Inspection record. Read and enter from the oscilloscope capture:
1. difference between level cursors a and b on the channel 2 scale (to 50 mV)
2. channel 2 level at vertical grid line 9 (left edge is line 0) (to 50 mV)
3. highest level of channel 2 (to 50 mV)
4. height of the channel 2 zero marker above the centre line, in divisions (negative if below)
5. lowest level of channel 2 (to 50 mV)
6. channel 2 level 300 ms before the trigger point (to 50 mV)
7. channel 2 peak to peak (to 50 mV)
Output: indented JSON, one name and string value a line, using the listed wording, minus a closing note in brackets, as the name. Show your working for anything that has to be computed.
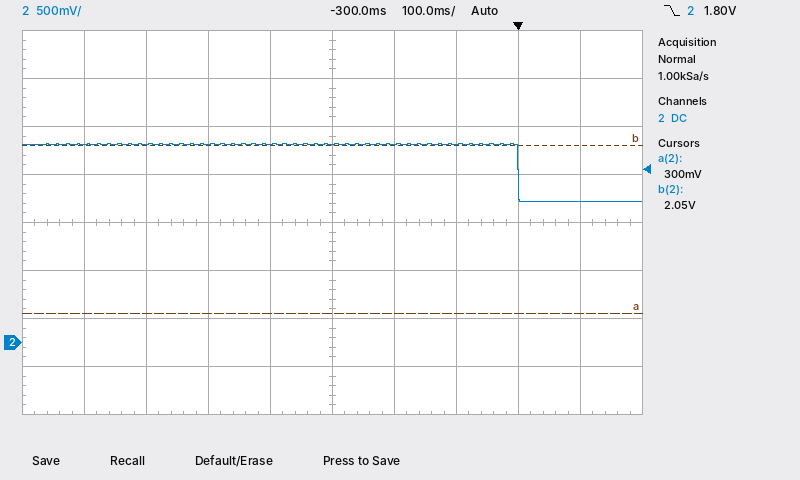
{
  "difference between level cursors a and b on the channel 2 scale": "1.75 V",
  "channel 2 level at vertical grid line 9 (left edge is line 0)": "1.45 V",
  "highest level of channel 2": "2.05 V",
  "height of the channel 2 zero marker above the centre line, in divisions": "-2.5 div",
  "lowest level of channel 2": "1.45 V",
  "channel 2 level 300 ms before the trigger point": "2.05 V",
  "channel 2 peak to peak": "2.05 V − (1.45 V) = 600 mV"
}
